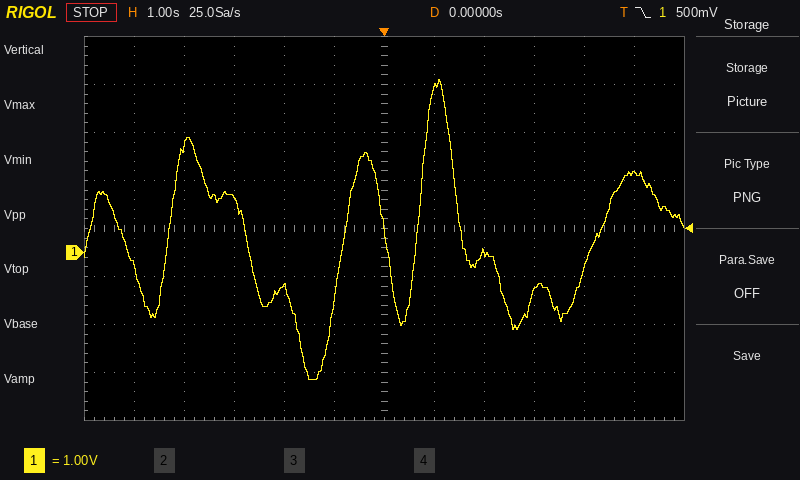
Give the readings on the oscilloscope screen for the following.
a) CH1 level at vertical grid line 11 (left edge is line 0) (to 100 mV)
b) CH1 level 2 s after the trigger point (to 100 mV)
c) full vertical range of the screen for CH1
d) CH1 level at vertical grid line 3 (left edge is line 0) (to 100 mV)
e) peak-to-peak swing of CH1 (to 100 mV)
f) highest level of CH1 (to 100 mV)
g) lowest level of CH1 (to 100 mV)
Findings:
1.6 V
0.0 V
8 V
1.1 V
6.2 V
3.6 V
-2.6 V
